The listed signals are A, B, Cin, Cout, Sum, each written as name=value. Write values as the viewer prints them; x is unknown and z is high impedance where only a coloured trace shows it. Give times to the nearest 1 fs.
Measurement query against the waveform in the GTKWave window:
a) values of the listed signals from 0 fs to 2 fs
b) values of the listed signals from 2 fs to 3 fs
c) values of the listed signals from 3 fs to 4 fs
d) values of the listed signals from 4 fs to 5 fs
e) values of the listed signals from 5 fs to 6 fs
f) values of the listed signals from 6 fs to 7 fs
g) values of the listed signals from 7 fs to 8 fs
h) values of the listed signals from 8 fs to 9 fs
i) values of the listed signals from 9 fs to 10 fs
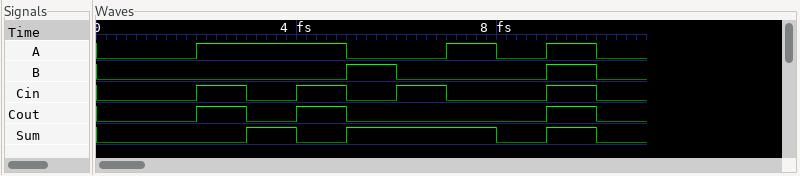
A=0, B=0, Cin=0, Cout=0, Sum=0
A=1, B=0, Cin=1, Cout=1, Sum=0
A=1, B=0, Cin=0, Cout=0, Sum=1
A=1, B=0, Cin=1, Cout=1, Sum=0
A=0, B=1, Cin=0, Cout=0, Sum=1
A=0, B=0, Cin=1, Cout=0, Sum=1
A=1, B=0, Cin=0, Cout=0, Sum=1
A=0, B=0, Cin=0, Cout=0, Sum=0
A=1, B=1, Cin=1, Cout=1, Sum=1
